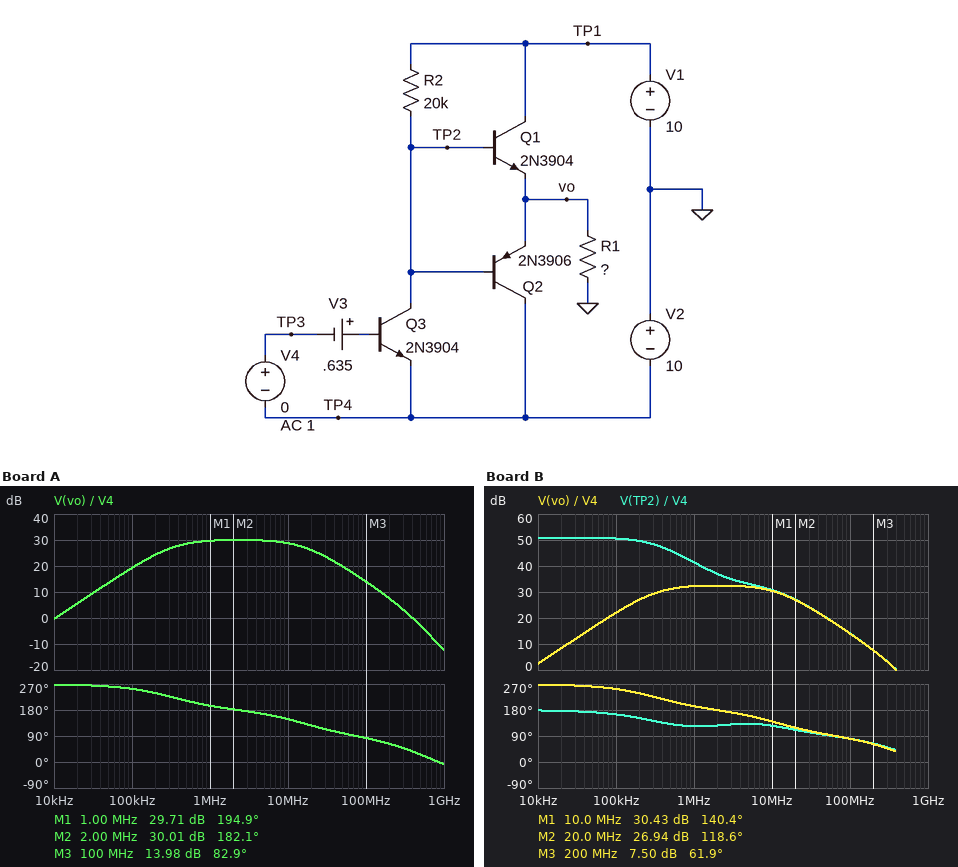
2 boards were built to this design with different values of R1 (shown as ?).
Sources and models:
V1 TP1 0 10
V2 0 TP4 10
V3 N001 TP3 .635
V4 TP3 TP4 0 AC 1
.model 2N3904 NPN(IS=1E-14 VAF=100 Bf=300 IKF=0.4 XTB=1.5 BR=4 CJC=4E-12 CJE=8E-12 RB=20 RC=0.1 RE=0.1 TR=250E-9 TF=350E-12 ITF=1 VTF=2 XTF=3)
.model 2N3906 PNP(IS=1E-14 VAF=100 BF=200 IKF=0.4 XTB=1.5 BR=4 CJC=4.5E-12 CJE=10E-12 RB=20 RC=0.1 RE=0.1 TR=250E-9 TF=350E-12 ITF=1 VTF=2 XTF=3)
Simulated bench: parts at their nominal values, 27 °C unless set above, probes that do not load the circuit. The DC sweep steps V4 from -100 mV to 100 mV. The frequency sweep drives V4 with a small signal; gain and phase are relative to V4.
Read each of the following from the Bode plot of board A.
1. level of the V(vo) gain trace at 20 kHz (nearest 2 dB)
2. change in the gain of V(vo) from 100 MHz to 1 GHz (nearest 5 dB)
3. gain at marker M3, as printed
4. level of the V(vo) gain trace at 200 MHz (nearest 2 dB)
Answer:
6 dB
-25 dB
13.98 dB
8 dB
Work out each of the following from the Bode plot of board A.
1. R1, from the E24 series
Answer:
2.4 kΩ
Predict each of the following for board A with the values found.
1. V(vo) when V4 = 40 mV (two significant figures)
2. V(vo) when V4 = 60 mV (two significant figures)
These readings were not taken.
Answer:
-9.3 V
-9.3 V
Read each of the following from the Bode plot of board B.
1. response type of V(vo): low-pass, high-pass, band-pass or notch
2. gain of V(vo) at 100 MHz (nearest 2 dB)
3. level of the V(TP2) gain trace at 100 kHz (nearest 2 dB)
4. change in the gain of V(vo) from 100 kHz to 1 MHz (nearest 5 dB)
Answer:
band-pass
14 dB
50 dB
10 dB
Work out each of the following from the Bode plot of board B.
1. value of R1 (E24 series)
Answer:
3.3 kΩ
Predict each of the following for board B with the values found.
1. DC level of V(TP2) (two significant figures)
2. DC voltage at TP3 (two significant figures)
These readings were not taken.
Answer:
-5.5 mV
-10 V
